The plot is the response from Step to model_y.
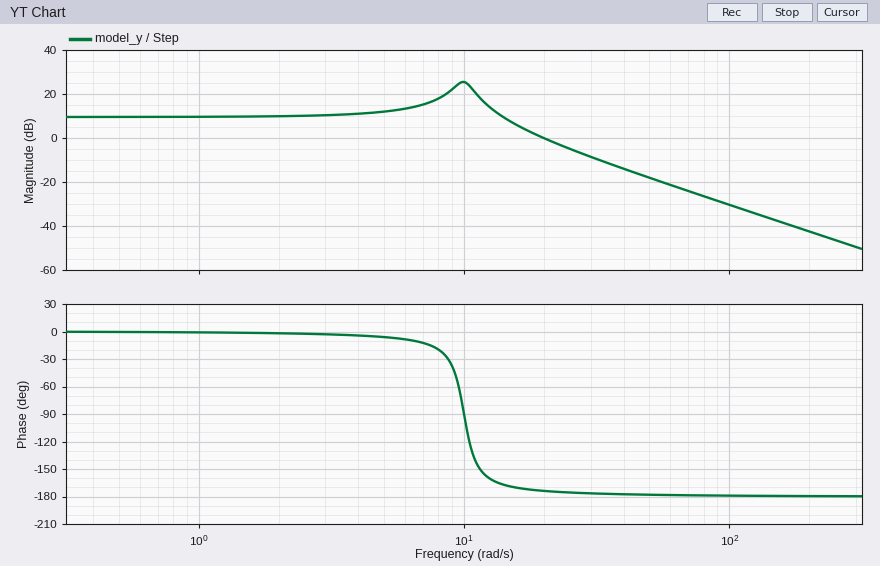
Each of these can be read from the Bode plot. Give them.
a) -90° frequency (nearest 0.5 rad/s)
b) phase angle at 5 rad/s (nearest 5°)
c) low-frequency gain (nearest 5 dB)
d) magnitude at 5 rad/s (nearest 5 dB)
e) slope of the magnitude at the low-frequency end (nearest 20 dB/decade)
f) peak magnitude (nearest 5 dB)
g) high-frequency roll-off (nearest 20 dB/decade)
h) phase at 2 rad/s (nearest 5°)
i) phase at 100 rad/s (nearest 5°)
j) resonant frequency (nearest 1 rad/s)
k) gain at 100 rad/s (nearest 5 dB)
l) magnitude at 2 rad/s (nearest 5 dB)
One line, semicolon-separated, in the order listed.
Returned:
10.0 rad/s; -5°; 10 dB; 10 dB; 0 dB/decade; 25 dB; -40 dB/decade; 0°; -180°; 10 rad/s; -30 dB; 10 dB
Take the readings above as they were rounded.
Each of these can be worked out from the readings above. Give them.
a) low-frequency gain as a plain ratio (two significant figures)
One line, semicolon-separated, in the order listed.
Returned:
3.2
